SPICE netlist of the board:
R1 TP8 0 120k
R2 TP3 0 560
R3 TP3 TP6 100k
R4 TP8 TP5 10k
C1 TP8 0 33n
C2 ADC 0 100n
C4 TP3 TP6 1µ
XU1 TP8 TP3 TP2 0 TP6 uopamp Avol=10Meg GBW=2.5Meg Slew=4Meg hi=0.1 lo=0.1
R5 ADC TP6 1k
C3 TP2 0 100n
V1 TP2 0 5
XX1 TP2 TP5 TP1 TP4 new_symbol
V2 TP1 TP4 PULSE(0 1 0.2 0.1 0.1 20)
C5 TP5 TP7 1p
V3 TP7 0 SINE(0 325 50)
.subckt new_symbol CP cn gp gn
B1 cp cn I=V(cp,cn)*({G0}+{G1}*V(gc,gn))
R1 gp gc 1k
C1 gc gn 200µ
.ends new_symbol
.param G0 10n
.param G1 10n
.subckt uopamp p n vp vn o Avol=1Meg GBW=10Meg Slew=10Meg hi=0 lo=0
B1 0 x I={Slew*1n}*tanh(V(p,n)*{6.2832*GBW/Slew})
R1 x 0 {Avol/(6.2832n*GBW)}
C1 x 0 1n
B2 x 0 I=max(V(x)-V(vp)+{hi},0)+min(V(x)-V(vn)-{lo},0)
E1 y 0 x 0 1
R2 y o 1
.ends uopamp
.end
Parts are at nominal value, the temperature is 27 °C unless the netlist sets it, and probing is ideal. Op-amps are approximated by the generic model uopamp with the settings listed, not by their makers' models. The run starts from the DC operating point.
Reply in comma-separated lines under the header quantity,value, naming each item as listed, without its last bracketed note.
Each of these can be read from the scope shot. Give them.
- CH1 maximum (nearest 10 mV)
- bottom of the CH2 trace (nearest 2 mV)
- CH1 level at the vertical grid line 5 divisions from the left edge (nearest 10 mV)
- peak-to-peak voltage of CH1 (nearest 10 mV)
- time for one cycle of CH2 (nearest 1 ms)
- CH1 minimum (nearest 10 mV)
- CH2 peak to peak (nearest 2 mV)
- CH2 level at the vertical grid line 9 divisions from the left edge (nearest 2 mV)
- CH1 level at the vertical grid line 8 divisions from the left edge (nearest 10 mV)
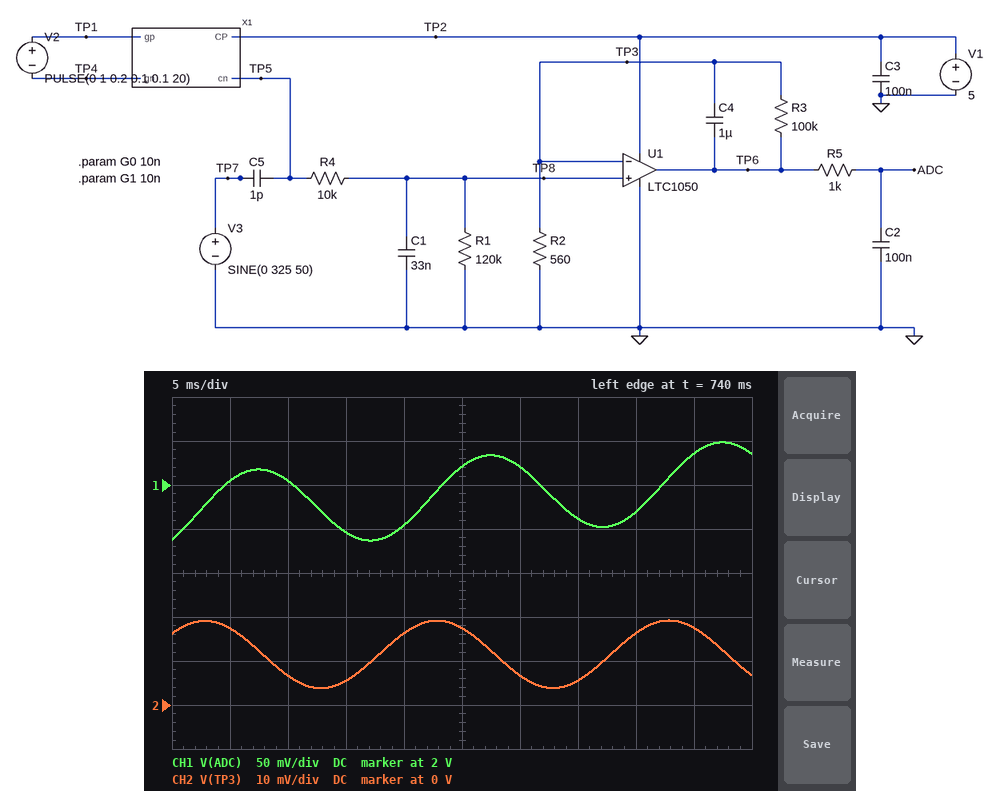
quantity,value
CH1 maximum,2.05 V
bottom of the CH2 trace,4 mV
CH1 level at the vertical grid line 5 divisions from the left edge,2.02 V
peak-to-peak voltage of CH1,110 mV
time for one cycle of CH2,20 ms
CH1 minimum,1.94 V
CH2 peak to peak,16 mV
CH2 level at the vertical grid line 9 divisions from the left edge,18 mV
CH1 level at the vertical grid line 8 divisions from the left edge,1.97 V
